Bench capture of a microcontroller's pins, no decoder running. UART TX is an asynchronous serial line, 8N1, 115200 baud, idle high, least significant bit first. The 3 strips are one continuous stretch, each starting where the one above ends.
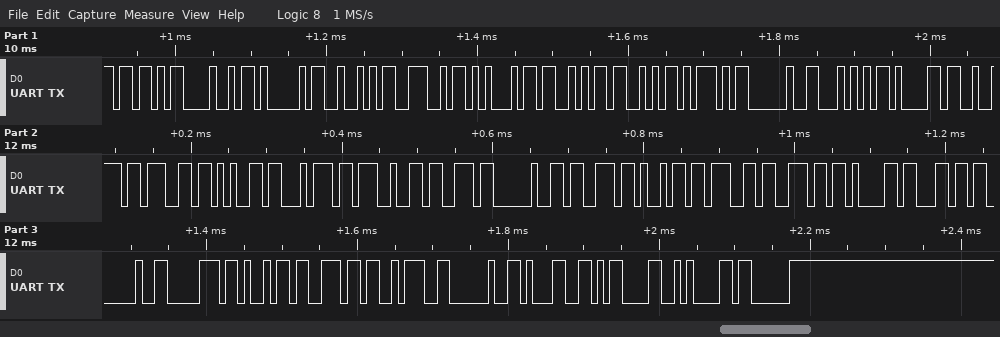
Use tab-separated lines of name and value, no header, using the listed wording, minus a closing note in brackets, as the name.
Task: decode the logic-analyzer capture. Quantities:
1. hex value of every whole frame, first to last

hex value of every whole frame, first to last	5B 48 41 52 4E 45 53 53 5D 20 54 61 72 67 65 74 27 73 20 73 69 67 6E 61 6C 20 70 69 6E 3A 20 31 0D 0A 03
